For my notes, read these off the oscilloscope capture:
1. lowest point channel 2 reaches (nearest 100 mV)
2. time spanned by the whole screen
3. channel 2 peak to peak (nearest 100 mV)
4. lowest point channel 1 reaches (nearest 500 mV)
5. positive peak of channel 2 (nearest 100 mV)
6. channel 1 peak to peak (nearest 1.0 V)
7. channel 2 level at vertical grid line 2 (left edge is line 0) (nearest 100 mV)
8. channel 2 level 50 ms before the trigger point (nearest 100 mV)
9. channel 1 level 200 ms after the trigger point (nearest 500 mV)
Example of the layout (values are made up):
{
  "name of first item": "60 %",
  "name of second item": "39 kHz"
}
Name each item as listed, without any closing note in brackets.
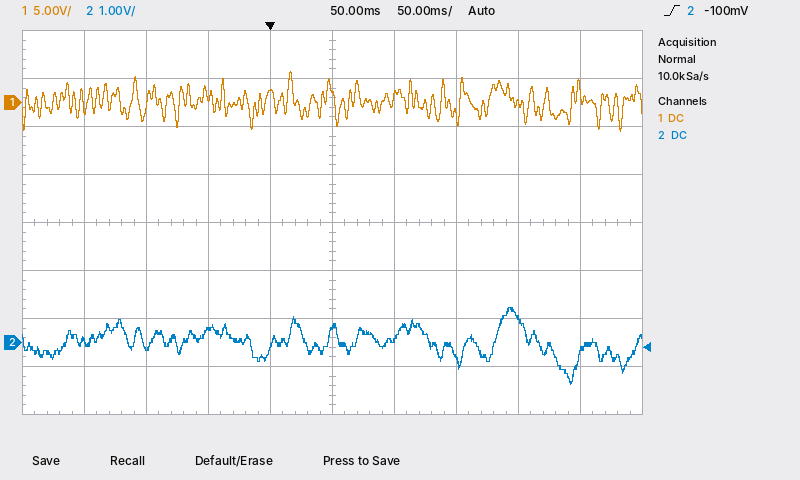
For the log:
{
  "lowest point channel 2 reaches": "-900 mV",
  "time spanned by the whole screen": "500 ms",
  "channel 2 peak to peak": "1.6 V",
  "lowest point channel 1 reaches": "-3.0 V",
  "positive peak of channel 2": "700 mV",
  "channel 1 peak to peak": "6.0 V",
  "channel 2 level at vertical grid line 2 (left edge is line 0)": "-100 mV",
  "channel 2 level 50 ms before the trigger point": "300 mV",
  "channel 1 level 200 ms after the trigger point": "0.0 V"
}
